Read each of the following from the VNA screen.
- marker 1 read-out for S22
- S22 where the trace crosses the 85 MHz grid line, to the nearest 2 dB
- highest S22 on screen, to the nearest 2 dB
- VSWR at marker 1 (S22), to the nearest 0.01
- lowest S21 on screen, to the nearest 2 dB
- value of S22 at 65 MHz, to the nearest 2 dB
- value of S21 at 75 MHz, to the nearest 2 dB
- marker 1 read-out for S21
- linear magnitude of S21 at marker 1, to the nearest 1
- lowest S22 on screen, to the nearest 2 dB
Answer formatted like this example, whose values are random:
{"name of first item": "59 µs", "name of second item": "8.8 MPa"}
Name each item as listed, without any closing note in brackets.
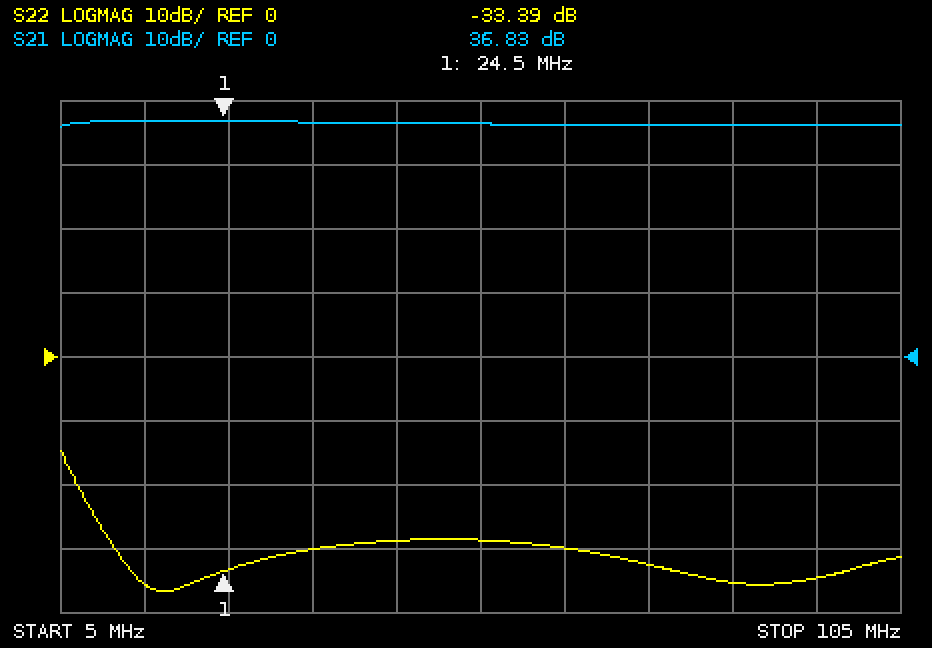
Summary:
{"marker 1 read-out for S22": "-33.39 dB", "S22 where the trace crosses the 85 MHz grid line, to the nearest 2 dB": "-36 dB", "highest S22 on screen, to the nearest 2 dB": "-14 dB", "VSWR at marker 1 (S22), to the nearest 0.01": "1.04", "lowest S21 on screen, to the nearest 2 dB": "36 dB", "value of S22 at 65 MHz, to the nearest 2 dB": "-30 dB", "value of S21 at 75 MHz, to the nearest 2 dB": "36 dB", "marker 1 read-out for S21": "36.83 dB", "linear magnitude of S21 at marker 1, to the nearest 1": "69", "lowest S22 on screen, to the nearest 2 dB": "-36 dB"}
